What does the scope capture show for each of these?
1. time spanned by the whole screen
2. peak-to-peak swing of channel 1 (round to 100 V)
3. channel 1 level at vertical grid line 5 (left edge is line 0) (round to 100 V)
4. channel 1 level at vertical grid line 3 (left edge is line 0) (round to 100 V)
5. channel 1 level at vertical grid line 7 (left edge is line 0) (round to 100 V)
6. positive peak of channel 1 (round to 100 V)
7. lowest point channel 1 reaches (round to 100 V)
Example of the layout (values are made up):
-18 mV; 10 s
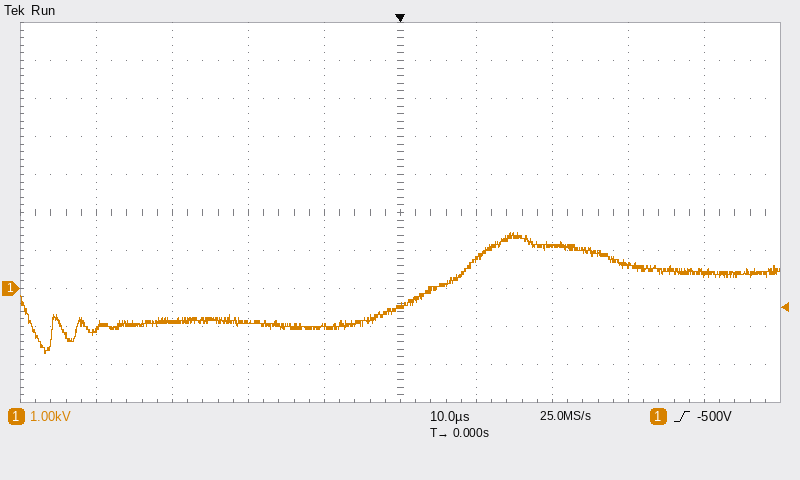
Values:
100 µs; 3.2 kV; -400 V; -900 V; 1.1 kV; 1.5 kV; -1.7 kV
